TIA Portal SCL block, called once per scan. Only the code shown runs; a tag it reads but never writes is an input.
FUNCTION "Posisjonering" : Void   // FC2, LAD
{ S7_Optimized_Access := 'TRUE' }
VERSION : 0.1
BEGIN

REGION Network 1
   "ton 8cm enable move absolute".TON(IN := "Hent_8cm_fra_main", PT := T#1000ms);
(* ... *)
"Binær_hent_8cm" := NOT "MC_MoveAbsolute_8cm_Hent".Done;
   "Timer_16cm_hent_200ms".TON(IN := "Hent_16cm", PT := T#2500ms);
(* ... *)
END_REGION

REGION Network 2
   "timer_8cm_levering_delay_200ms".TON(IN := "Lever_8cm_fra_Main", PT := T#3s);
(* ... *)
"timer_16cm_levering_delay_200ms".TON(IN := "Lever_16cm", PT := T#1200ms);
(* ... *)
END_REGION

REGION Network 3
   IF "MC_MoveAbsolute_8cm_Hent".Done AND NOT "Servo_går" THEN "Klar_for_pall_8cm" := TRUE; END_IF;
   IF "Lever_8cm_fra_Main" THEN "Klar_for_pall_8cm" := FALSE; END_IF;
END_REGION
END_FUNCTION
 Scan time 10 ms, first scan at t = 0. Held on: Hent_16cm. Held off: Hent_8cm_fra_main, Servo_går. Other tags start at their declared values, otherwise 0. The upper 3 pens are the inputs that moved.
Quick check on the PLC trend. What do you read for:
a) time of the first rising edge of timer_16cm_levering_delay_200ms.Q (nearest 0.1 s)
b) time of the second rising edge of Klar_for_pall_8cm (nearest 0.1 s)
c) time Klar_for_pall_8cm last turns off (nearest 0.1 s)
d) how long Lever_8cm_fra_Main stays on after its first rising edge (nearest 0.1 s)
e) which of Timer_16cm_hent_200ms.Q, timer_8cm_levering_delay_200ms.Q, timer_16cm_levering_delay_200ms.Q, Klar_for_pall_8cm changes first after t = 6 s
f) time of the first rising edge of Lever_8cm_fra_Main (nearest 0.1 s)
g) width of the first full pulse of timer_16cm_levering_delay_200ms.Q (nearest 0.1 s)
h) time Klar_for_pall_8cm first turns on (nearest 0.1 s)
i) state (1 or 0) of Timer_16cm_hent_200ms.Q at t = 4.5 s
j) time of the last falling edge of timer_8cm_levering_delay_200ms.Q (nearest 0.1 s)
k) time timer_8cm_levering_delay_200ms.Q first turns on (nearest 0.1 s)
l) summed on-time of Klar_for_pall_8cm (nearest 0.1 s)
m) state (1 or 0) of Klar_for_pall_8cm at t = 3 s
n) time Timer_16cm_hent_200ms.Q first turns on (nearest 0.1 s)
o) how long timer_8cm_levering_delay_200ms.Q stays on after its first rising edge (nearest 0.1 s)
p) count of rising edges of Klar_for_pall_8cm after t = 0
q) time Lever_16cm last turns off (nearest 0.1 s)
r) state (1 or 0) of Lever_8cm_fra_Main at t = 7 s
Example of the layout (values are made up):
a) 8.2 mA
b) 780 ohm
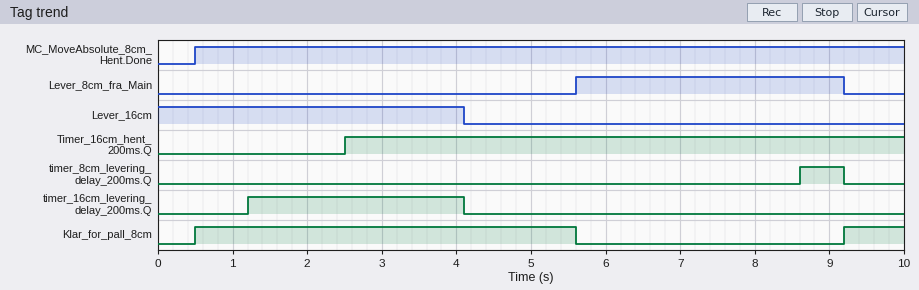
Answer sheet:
a) 1.2 s
b) 9.2 s
c) 5.6 s
d) 3.6 s
e) timer_8cm_levering_delay_200ms.Q
f) 5.6 s
g) 2.9 s
h) 0.5 s
i) 1
j) 9.2 s
k) 8.6 s
l) 5.9 s
m) 1
n) 2.5 s
o) 0.6 s
p) 2
q) 4.1 s
r) 1
